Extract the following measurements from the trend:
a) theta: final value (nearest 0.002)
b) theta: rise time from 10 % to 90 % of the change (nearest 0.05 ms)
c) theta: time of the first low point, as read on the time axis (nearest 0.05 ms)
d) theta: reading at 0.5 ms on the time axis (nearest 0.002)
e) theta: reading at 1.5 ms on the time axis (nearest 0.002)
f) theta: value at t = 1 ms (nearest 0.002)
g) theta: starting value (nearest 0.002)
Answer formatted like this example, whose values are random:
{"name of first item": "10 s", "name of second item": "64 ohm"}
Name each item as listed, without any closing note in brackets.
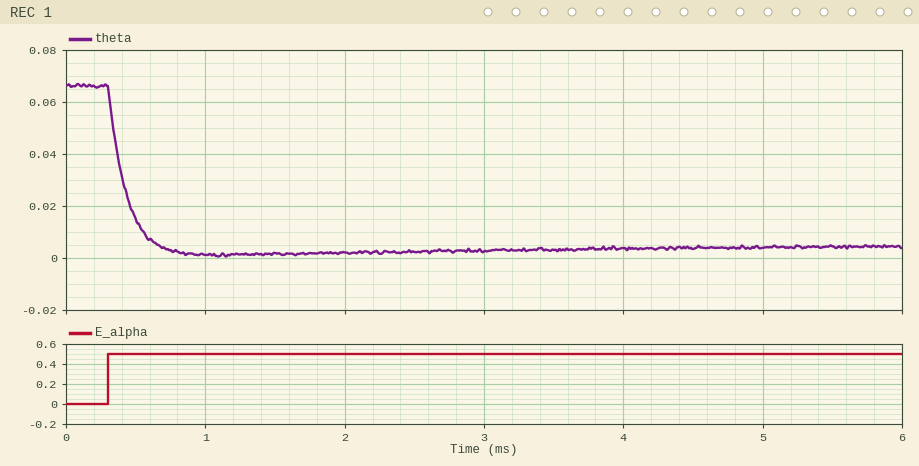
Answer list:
{"theta: final value": "0.004", "theta: rise time from 10 % to 90 % of the change": "0.25 ms", "theta: time of the first low point, as read on the time axis": "1.10 ms", "theta: reading at 0.5 ms on the time axis": "0.016", "theta: reading at 1.5 ms on the time axis": "0.002", "theta: value at t = 1 ms": "0.002", "theta: starting value": "0.066"}
